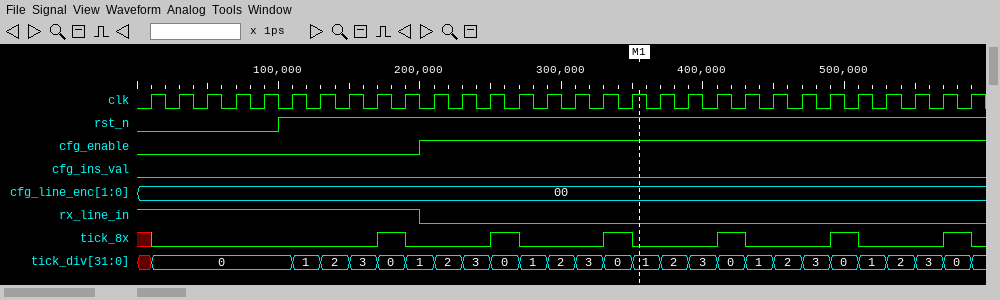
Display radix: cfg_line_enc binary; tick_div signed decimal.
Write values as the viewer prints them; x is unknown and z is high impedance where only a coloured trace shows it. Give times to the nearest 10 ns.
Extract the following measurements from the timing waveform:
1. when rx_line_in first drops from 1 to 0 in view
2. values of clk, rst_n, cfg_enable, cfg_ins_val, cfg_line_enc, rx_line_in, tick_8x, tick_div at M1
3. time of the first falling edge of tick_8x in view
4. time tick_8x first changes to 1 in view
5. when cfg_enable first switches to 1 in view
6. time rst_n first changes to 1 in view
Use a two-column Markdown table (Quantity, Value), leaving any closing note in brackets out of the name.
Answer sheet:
| Quantity | Value |
|---|---|
| when rx_line_in first drops from 1 to 0 in view | 200 ns |
| values of clk, rst_n, cfg_enable, cfg_ins_val, cfg_line_enc, rx_line_in, tick_8x, tick_div at M1 | clk=1, rst_n=1, cfg_enable=1, cfg_ins_val=0, cfg_line_enc=00, rx_line_in=0, tick_8x=0, tick_div=1 |
| time of the first falling edge of tick_8x in view | 190 ns |
| time tick_8x first changes to 1 in view | 170 ns |
| when cfg_enable first switches to 1 in view | 200 ns |
| time rst_n first changes to 1 in view | 100 ns |
